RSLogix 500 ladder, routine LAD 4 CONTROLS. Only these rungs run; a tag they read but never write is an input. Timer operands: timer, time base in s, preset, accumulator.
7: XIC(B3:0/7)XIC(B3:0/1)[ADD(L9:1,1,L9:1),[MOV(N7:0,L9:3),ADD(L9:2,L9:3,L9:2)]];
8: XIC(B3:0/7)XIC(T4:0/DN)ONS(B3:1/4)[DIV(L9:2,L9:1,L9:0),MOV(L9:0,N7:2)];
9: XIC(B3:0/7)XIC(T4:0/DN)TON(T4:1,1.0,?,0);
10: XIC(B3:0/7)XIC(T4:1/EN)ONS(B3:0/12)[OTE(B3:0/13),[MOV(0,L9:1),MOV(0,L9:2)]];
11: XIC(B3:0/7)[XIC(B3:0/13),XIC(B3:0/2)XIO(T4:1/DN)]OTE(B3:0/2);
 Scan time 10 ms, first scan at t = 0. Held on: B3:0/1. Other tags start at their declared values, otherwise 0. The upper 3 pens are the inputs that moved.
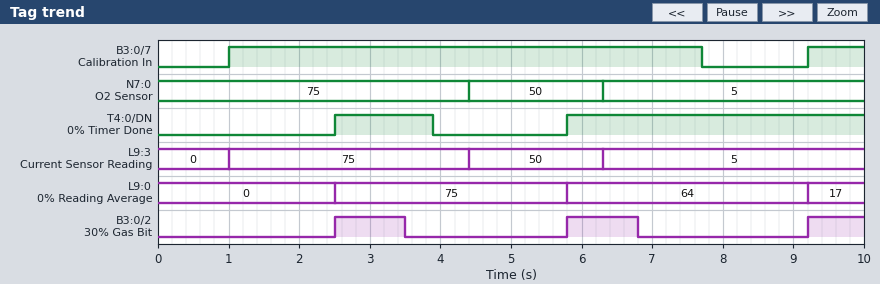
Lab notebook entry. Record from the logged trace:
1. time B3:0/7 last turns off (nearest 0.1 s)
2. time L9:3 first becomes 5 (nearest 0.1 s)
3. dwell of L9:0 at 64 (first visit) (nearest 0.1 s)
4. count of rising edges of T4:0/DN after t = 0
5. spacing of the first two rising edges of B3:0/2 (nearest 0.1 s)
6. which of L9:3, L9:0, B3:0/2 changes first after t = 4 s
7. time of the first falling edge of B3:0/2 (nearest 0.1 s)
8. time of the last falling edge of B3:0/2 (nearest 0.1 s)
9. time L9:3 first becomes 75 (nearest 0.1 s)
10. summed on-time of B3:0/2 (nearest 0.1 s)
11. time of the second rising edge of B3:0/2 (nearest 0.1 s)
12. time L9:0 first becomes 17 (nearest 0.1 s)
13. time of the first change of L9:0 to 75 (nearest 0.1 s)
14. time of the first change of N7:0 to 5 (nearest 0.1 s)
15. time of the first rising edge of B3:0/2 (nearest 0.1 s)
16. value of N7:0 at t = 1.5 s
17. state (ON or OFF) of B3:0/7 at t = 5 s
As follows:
7.7 s
6.3 s
3.4 s
2
3.3 s
L9:3
3.5 s
6.8 s
1.0 s
2.8 s
5.8 s
9.2 s
2.5 s
6.3 s
2.5 s
75
ON
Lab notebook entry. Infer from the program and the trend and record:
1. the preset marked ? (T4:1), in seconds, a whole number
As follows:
1 s
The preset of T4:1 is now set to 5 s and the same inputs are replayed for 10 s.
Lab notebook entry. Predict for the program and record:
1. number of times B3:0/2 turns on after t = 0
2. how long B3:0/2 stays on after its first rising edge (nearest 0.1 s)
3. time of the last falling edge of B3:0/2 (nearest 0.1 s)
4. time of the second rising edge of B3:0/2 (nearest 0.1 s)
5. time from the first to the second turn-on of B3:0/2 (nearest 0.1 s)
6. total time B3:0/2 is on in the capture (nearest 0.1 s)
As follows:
2
5.2 s
7.7 s
9.2 s
6.7 s
6.0 s
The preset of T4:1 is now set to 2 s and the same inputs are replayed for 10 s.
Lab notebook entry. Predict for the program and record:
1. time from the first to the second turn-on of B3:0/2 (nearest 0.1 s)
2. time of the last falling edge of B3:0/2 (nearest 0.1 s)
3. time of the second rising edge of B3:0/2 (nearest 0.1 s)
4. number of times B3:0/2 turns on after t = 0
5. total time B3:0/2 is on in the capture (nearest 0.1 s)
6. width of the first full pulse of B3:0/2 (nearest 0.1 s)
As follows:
6.7 s
7.7 s
9.2 s
2
6.0 s
5.2 s
